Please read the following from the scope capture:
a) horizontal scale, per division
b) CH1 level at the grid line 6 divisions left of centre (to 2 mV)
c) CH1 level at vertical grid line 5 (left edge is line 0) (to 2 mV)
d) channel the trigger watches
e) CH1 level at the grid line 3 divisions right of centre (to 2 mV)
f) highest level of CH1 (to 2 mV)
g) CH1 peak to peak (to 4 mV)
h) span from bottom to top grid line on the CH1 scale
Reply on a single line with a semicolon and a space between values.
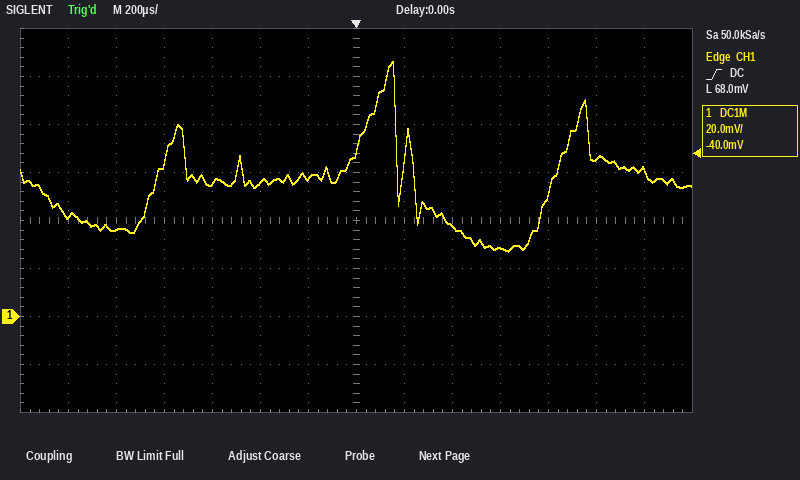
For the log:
200 µs; 42 mV; 56 mV; CH1; 28 mV; 106 mV; 80 mV; 160 mV
